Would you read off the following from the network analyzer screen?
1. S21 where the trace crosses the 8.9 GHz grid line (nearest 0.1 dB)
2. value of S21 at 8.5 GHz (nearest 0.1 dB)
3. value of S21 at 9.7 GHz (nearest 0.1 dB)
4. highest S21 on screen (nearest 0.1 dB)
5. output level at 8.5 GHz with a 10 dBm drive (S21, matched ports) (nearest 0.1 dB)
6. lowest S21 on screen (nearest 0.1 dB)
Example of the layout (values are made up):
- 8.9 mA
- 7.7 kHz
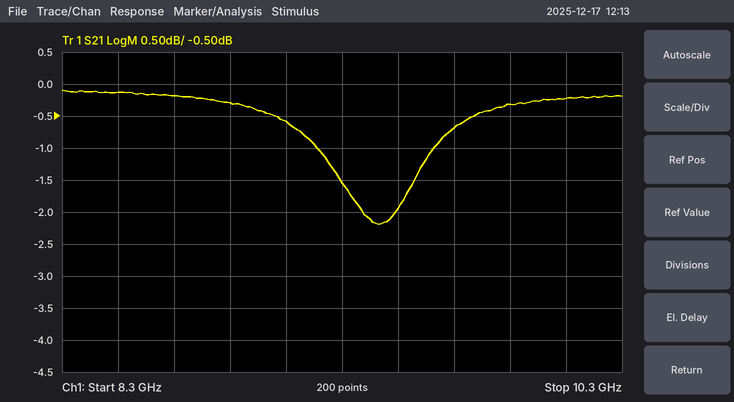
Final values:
- -0.3 dB
- -0.1 dB
- -0.7 dB
- -0.1 dB
- 9.9 dBm
- -2.2 dB
